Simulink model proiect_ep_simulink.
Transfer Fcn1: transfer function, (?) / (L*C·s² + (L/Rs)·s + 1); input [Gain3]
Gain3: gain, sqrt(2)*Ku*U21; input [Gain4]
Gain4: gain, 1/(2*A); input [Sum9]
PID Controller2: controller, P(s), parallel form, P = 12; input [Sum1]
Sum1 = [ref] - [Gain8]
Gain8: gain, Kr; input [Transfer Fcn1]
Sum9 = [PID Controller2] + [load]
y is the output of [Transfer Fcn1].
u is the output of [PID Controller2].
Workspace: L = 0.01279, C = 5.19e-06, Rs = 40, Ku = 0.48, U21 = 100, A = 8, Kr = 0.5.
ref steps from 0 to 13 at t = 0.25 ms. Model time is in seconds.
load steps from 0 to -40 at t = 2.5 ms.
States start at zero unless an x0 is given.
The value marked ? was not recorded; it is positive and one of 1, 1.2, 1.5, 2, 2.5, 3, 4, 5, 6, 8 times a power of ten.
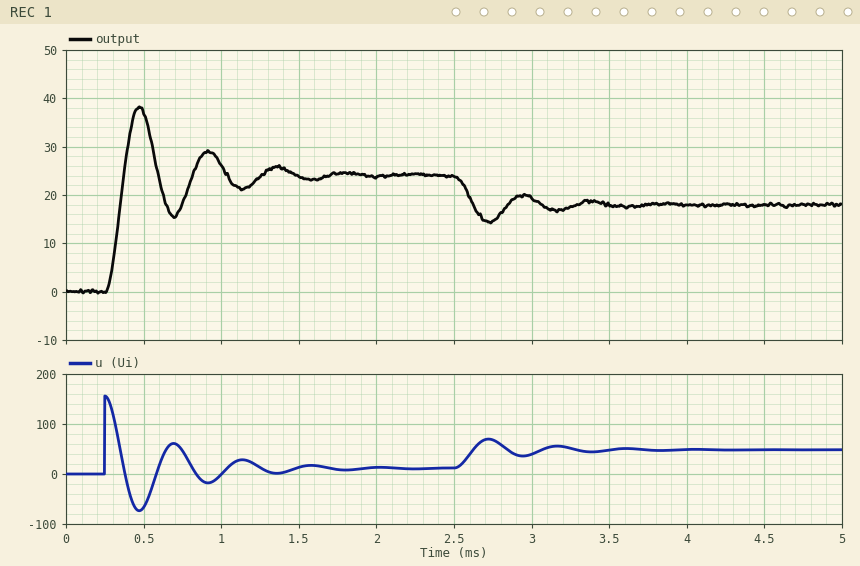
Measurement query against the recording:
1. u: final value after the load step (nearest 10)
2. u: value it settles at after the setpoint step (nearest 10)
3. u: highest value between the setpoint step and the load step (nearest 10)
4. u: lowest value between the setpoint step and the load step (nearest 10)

50
10
160
-70
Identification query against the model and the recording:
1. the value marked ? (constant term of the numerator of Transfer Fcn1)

0.5
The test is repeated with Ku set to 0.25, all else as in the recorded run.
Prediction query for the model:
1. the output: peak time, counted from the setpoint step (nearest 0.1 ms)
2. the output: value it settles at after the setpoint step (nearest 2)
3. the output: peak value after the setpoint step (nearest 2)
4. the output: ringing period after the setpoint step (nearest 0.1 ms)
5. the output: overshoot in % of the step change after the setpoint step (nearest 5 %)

0.3 ms
22
34
0.6 ms
50 %
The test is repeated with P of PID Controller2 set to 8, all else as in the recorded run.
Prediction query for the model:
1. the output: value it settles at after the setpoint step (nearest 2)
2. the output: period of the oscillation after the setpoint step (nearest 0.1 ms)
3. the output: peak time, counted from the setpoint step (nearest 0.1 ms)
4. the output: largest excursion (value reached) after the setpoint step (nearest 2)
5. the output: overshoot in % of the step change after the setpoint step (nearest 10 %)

24
0.5 ms
0.3 ms
36
50 %
